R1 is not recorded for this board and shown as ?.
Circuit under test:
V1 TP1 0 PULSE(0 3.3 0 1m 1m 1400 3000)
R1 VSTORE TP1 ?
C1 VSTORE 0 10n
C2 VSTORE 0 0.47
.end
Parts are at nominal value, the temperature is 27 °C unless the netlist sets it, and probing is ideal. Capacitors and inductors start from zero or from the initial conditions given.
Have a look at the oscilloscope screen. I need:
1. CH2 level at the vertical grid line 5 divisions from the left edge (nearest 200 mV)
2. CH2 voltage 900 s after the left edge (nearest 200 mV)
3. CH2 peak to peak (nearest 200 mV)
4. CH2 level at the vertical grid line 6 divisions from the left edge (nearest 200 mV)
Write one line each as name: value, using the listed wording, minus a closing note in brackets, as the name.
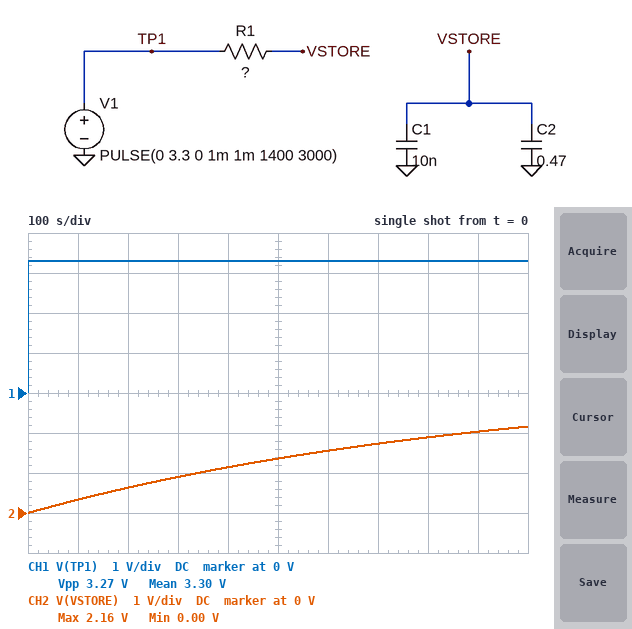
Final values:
CH2 level at the vertical grid line 5 divisions from the left edge: 1.4 V
CH2 voltage 900 s after the left edge: 2.0 V
CH2 peak to peak: 2.2 V
CH2 level at the vertical grid line 6 divisions from the left edge: 1.6 V
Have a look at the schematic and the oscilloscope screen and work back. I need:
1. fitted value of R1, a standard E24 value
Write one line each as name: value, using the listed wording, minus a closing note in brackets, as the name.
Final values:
fitted value of R1, a standard E24 value: 2 kΩ
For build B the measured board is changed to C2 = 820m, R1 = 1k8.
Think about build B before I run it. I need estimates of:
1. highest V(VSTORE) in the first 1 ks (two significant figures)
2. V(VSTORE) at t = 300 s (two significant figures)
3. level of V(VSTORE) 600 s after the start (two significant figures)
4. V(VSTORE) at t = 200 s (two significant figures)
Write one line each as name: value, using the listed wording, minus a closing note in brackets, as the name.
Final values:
highest V(VSTORE) in the first 1 ks: 1.6 V
V(VSTORE) at t = 300 s: 610 mV
level of V(VSTORE) 600 s after the start: 1.1 V
V(VSTORE) at t = 200 s: 420 mV
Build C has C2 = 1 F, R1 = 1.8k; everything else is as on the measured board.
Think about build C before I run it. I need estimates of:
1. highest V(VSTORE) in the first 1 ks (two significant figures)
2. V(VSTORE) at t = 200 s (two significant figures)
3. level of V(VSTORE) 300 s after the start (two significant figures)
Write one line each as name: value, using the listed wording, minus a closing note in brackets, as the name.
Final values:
highest V(VSTORE) in the first 1 ks: 1.4 V
V(VSTORE) at t = 200 s: 350 mV
level of V(VSTORE) 300 s after the start: 510 mV
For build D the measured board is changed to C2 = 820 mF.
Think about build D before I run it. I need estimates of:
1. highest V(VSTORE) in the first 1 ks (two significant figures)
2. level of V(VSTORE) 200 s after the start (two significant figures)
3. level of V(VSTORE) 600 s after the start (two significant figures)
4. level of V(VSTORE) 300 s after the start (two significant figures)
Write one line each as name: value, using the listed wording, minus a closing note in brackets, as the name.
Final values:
highest V(VSTORE) in the first 1 ks: 1.5 V
level of V(VSTORE) 200 s after the start: 380 mV
level of V(VSTORE) 600 s after the start: 1.0 V
level of V(VSTORE) 300 s after the start: 550 mV
